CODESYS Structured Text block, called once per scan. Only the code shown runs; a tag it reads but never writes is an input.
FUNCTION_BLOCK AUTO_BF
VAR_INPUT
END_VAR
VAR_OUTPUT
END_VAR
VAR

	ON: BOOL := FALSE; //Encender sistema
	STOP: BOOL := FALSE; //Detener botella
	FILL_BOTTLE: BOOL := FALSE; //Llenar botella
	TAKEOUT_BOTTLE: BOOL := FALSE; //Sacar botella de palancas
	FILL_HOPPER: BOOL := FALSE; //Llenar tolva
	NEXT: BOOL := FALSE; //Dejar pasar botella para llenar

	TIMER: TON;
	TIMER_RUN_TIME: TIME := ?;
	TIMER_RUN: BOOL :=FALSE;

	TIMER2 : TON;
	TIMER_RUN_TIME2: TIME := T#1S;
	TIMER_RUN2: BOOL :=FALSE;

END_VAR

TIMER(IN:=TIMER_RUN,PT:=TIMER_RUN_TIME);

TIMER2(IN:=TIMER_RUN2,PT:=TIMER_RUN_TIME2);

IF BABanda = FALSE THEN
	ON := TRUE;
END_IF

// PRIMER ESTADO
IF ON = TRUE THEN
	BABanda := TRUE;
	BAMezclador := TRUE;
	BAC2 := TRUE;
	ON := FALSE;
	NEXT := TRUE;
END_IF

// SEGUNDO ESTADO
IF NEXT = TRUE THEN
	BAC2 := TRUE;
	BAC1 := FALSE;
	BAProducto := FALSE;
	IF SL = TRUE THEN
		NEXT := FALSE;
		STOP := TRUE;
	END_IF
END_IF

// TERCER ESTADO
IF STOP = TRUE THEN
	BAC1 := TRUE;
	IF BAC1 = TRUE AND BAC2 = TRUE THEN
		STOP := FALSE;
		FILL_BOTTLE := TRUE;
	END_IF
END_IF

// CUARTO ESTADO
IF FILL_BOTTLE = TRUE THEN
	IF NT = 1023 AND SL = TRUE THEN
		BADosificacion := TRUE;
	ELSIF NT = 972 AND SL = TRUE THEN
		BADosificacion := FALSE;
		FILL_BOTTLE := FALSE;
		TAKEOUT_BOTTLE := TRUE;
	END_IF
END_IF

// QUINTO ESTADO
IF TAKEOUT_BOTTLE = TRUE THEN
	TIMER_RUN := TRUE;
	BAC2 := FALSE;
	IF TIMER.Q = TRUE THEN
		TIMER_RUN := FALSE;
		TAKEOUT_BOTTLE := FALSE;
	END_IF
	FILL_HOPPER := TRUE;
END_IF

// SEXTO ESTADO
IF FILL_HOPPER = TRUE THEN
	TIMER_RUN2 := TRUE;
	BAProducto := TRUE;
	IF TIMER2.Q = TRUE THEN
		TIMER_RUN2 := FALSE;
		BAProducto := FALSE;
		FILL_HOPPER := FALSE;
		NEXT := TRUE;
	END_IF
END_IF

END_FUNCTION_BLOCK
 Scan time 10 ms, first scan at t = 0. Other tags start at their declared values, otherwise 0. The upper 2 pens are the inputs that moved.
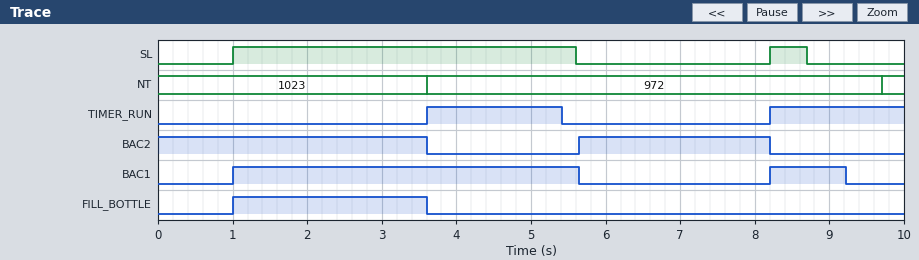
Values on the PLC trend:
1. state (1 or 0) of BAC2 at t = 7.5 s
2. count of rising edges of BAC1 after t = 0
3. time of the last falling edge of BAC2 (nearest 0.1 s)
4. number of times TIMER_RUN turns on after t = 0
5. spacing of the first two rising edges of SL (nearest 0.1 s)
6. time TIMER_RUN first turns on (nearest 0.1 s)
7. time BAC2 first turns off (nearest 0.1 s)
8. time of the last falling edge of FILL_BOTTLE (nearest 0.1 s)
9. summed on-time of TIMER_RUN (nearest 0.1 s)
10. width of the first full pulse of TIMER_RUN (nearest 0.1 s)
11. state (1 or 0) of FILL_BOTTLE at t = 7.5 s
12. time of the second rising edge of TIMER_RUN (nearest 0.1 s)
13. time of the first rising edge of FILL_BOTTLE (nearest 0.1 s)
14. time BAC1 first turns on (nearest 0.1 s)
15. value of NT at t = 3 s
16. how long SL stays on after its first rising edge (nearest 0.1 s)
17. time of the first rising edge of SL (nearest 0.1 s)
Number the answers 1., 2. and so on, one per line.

1. 1
2. 2
3. 8.2 s
4. 2
5. 7.2 s
6. 3.6 s
7. 3.6 s
8. 3.6 s
9. 3.6 s
10. 1.8 s
11. 0
12. 8.2 s
13. 1.0 s
14. 1.0 s
15. 1023
16. 4.6 s
17. 1.0 s
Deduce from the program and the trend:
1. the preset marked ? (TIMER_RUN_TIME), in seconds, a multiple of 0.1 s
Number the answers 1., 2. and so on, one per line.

1. 1.8 s
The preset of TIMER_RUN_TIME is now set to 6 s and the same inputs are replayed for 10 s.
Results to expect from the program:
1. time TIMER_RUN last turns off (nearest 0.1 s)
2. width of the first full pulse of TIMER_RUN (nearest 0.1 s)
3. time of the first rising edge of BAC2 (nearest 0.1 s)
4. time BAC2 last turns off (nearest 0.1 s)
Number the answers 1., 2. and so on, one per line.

1. 9.6 s
2. 6.0 s
3. 9.6 s
4. 3.6 s
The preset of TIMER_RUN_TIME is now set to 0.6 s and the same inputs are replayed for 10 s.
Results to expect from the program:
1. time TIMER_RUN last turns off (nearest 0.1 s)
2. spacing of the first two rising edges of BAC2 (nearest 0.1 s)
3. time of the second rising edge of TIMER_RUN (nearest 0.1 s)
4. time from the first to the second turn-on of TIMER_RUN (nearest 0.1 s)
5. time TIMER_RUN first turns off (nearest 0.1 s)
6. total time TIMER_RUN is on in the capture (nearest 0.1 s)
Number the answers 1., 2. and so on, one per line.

1. 8.8 s
2. 3.6 s
3. 4.6 s
4. 1.0 s
5. 4.2 s
6. 1.8 s
